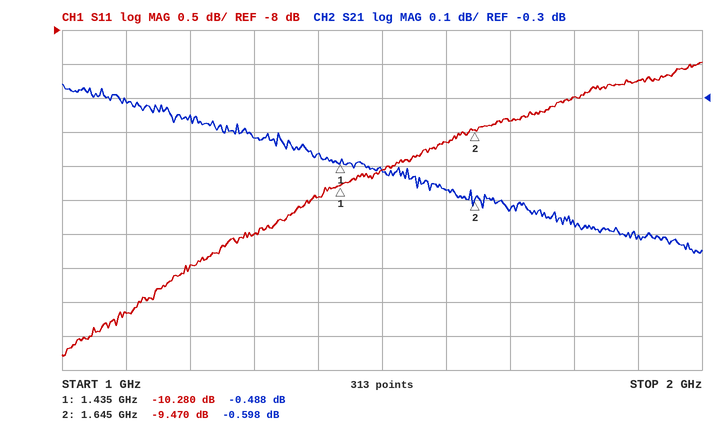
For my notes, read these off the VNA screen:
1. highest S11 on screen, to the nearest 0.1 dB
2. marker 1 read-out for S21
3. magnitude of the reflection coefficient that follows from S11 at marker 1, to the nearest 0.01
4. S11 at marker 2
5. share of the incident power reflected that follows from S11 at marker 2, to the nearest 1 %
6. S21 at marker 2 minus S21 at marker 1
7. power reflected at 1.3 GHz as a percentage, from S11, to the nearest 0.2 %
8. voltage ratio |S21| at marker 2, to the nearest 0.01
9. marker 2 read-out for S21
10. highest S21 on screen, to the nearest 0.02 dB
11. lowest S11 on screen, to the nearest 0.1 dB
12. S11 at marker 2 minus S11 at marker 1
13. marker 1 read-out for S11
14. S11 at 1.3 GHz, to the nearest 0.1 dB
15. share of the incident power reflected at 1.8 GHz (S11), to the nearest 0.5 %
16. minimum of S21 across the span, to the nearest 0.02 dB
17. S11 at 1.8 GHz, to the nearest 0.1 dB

-8.5 dB
-0.488 dB
0.31
-9.470 dB
11 %
-0.110 dB
8.0 %
0.93
-0.598 dB
-0.26 dB
-12.8 dB
0.810 dB
-10.280 dB
-11.0 dB
12.5 %
-0.76 dB
-9.0 dB
